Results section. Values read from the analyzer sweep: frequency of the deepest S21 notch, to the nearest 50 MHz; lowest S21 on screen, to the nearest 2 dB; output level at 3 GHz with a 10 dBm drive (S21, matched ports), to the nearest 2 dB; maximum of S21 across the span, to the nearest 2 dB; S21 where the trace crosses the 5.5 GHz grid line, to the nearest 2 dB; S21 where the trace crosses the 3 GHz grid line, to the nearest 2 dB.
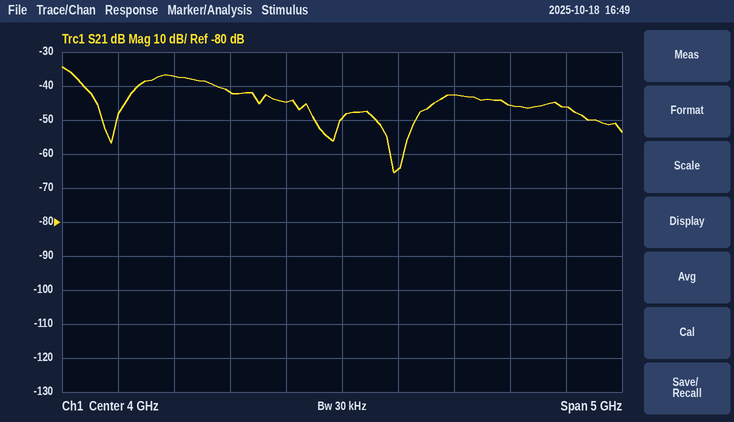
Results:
4.45 GHz
-66 dB
-32 dBm
-34 dB
-46 dB
-42 dB
